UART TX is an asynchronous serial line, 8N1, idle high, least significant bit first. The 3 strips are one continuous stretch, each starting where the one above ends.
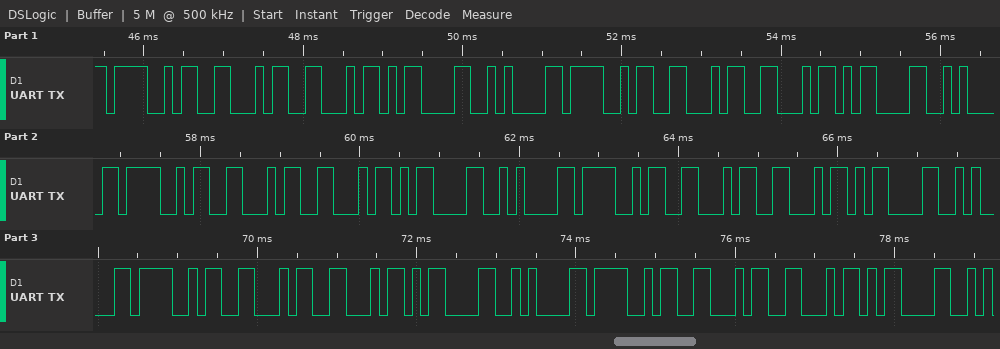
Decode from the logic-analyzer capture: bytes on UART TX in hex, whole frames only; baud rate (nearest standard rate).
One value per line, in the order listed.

4F 46 46 0D 0A 4F 46 46 0D 0A 4F 46 46 0D 0A 4F 46 46 0D 0A 4F 46 46 0D 0A 4F 46 46 0D
9600 baud
